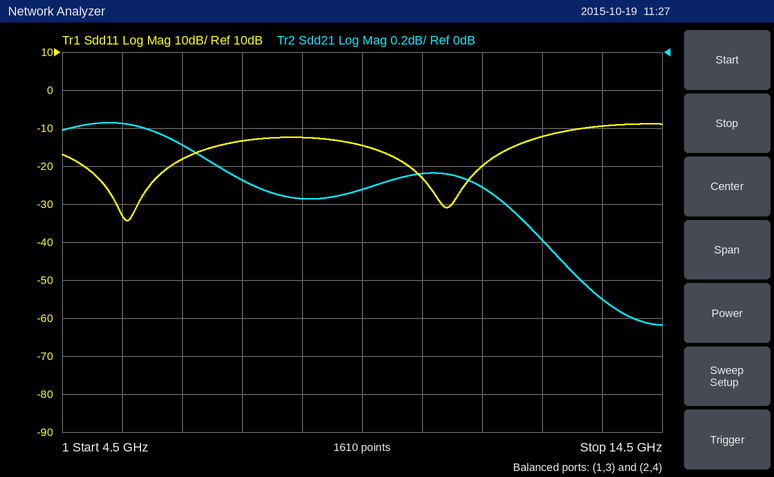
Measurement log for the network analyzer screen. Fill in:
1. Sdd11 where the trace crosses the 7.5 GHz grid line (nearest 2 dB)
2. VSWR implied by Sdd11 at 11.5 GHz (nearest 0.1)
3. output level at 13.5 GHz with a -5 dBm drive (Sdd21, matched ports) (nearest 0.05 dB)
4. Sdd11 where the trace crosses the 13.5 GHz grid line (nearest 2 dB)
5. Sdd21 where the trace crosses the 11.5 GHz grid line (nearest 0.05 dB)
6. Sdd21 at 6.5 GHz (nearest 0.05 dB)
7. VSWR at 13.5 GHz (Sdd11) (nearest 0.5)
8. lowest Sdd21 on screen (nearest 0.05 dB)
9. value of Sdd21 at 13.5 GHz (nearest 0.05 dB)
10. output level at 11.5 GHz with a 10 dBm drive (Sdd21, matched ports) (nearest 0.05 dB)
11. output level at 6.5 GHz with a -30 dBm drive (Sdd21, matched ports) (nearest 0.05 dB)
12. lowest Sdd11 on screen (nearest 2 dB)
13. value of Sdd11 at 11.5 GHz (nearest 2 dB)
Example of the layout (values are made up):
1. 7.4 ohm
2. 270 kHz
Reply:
1. -14 dB
2. 1.2
3. -6.30 dBm
4. -10 dB
5. -0.70 dB
6. -0.50 dB
7. 2.0
8. -1.45 dB
9. -1.30 dB
10. 9.30 dBm
11. -30.50 dBm
12. -34 dB
13. -20 dB
